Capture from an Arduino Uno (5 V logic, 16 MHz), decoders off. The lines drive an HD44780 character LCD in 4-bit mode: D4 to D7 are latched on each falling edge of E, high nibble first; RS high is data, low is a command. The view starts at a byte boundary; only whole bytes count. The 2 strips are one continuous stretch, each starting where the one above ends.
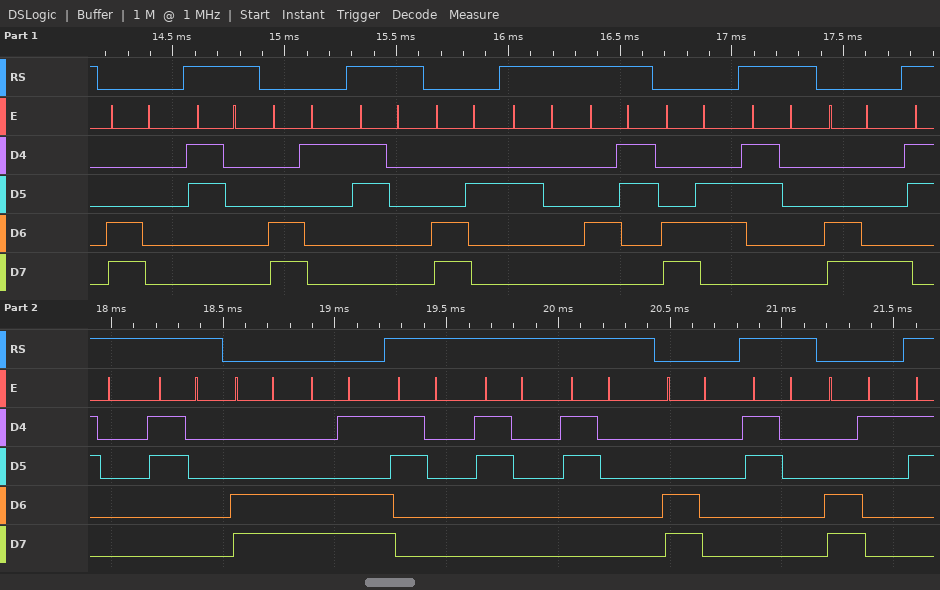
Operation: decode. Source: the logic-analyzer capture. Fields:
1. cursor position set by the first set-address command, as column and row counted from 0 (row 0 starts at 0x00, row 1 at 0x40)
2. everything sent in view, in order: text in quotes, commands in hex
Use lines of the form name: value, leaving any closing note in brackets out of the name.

cursor position set by the first set-address command, as column and row counted from 0: column 0, row 1
everything sent in view, in order: text in quotes, commands in hex: 0xC0 "0" 0xC1 "0" 0xC2 " C" 0xC6 "0" 0xC8 "00" 0xCC 0xCD "000" 0xC0 "0" 0xC1
